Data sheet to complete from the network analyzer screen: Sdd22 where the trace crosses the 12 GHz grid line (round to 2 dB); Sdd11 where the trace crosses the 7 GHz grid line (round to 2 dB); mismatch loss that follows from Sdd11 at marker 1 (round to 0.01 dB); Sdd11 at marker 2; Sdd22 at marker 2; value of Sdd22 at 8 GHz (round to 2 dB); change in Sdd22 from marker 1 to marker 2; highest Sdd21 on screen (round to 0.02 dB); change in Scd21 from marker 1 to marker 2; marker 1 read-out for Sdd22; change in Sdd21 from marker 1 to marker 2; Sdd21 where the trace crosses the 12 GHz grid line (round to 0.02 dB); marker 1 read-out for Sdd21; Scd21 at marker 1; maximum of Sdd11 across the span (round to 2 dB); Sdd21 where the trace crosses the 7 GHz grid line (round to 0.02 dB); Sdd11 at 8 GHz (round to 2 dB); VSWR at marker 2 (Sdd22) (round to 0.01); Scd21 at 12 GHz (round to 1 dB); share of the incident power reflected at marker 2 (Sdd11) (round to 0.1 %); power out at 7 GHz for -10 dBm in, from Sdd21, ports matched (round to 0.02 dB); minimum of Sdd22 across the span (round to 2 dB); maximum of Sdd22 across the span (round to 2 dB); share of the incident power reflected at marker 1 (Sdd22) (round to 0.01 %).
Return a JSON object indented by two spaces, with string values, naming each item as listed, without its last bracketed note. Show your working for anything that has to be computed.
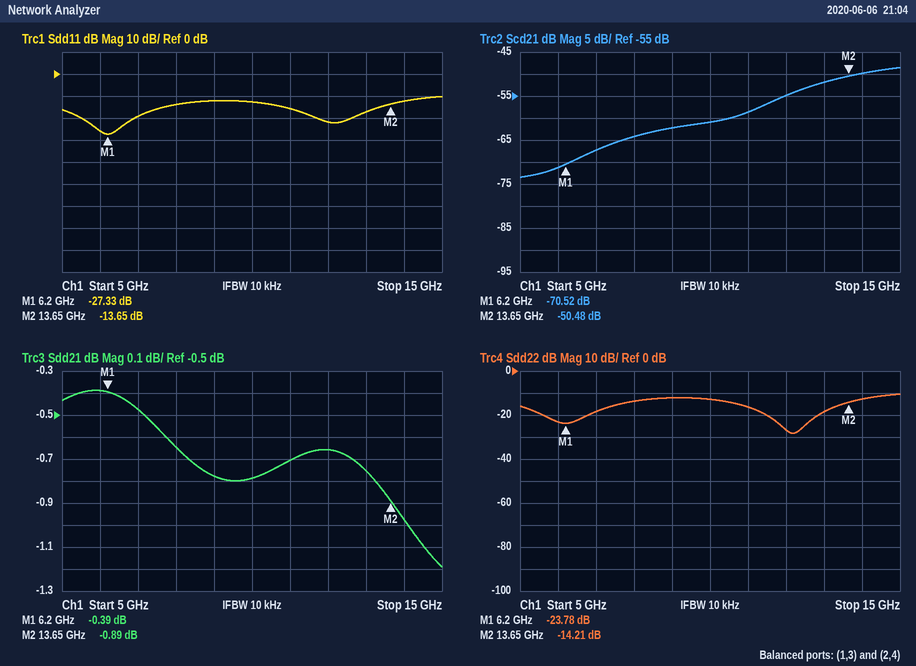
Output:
{
  "Sdd22 where the trace crosses the 12 GHz grid line": "-26 dB",
  "Sdd11 where the trace crosses the 7 GHz grid line": "-20 dB",
  "mismatch loss that follows from Sdd11 at marker 1": "−10 log10(1 − 10^(-27.33/10)) ≈ 0.01 dB",
  "Sdd11 at marker 2": "-13.65 dB",
  "Sdd22 at marker 2": "-14.21 dB",
  "value of Sdd22 at 8 GHz": "-14 dB",
  "change in Sdd22 from marker 1 to marker 2": "-14.21 − (-23.78) = 9.57 dB",
  "highest Sdd21 on screen": "-0.38 dB",
  "change in Scd21 from marker 1 to marker 2": "-50.48 − (-70.52) = 20.04 dB",
  "marker 1 read-out for Sdd22": "-23.78 dB",
  "change in Sdd21 from marker 1 to marker 2": "-0.89 − (-0.39) = -0.50 dB",
  "Sdd21 where the trace crosses the 12 GHz grid line": "-0.66 dB",
  "marker 1 read-out for Sdd21": "-0.39 dB",
  "Scd21 at marker 1": "-70.52 dB",
  "maximum of Sdd11 across the span": "-10 dB",
  "Sdd21 where the trace crosses the 7 GHz grid line": "-0.48 dB",
  "Sdd11 at 8 GHz": "-14 dB",
  "VSWR at marker 2 (Sdd22)": "(1 + 0.1948)/(1 − 0.1948) ≈ 1.48",
  "Scd21 at 12 GHz": "-55 dB",
  "share of the incident power reflected at marker 2 (Sdd11)": "10^(-13.65/10) ≈ 4.3 %",
  "power out at 7 GHz for -10 dBm in, from Sdd21, ports matched": "-10 dBm + (-0.48 dB) = -10.48 dBm",
  "minimum of Sdd22 across the span": "-28 dB",
  "maximum of Sdd22 across the span": "-10 dB",
  "share of the incident power reflected at marker 1 (Sdd22)": "10^(-23.78/10) ≈ 0.42 %"
}
